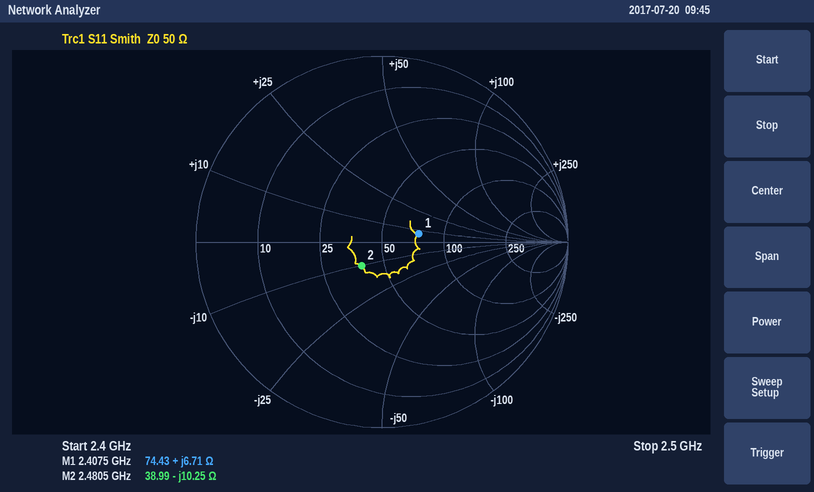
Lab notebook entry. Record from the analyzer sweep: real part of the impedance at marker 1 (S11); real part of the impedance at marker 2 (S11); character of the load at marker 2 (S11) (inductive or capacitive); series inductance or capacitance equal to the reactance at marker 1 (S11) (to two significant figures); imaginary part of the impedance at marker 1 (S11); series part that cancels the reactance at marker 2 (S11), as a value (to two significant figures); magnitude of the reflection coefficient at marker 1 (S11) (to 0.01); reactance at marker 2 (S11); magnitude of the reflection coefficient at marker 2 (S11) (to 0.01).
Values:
74.43 Ω
38.99 Ω
capacitive
440 pH
+6.71 Ω
660 pH
0.20
-10.25 Ω
0.17
